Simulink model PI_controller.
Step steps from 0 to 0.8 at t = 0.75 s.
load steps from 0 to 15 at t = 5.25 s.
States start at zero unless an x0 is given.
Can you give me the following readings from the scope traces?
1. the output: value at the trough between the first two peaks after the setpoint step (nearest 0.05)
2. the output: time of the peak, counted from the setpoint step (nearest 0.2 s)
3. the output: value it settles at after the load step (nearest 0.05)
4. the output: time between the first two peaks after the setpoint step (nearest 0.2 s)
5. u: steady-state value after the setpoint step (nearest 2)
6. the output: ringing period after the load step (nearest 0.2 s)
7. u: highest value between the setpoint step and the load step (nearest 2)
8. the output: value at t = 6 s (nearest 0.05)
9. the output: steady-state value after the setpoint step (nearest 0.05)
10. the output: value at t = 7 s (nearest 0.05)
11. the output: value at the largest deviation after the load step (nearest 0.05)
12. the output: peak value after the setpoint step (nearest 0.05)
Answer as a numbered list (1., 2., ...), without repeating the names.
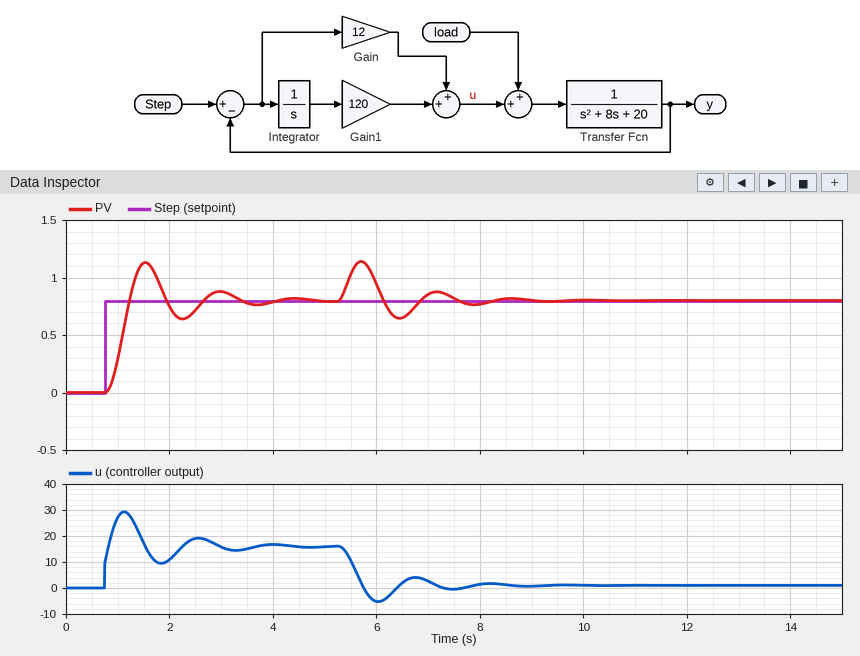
1. 0.65
2. 0.8 s
3. 0.80
4. 1.4 s
5. 16
6. 1.4 s
7. 30
8. 0.95
9. 0.80
10. 0.85
11. 1.15
12. 1.15
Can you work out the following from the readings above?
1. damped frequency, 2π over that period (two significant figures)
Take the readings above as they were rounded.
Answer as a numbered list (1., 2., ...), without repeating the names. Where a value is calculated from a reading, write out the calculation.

1. 2π / 1.4 = 4.5 rad/s
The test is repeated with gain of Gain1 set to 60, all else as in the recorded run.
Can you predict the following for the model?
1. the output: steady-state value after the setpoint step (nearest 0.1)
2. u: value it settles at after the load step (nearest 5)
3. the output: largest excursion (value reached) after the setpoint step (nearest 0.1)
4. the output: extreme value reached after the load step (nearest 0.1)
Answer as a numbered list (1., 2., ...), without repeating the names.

1. 0.8
2. 0
3. 0.9
4. 1.2
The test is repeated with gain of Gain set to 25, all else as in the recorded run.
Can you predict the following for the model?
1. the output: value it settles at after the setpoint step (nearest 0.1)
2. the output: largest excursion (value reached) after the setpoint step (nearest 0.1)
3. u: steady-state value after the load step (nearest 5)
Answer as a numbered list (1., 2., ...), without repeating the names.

1. 0.8
2. 1.0
3. 0
